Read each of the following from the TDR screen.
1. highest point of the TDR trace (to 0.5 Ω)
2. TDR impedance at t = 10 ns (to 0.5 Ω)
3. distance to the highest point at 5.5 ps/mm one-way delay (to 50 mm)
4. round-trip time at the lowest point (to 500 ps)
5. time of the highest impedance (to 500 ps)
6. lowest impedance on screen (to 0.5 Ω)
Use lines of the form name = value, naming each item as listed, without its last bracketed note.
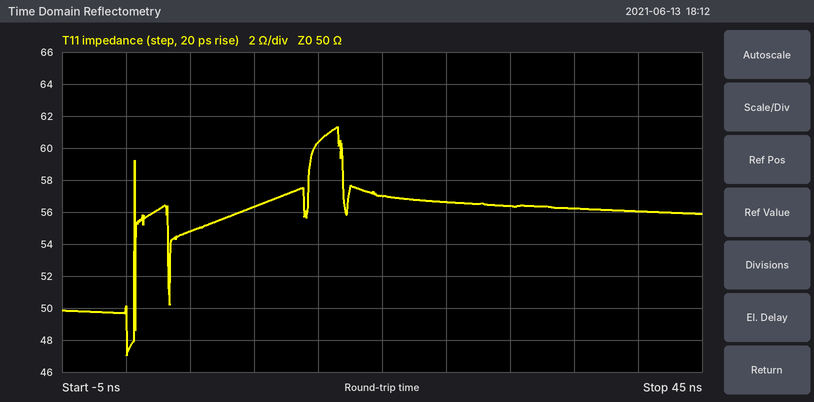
highest point of the TDR trace = 61.5 Ω
TDR impedance at t = 10 ns = 56.5 Ω
distance to the highest point at 5.5 ps/mm one-way delay = 1.50 m
round-trip time at the lowest point = 0.0 ns
time of the highest impedance = 16.5 ns
lowest impedance on screen = 47.0 Ω
